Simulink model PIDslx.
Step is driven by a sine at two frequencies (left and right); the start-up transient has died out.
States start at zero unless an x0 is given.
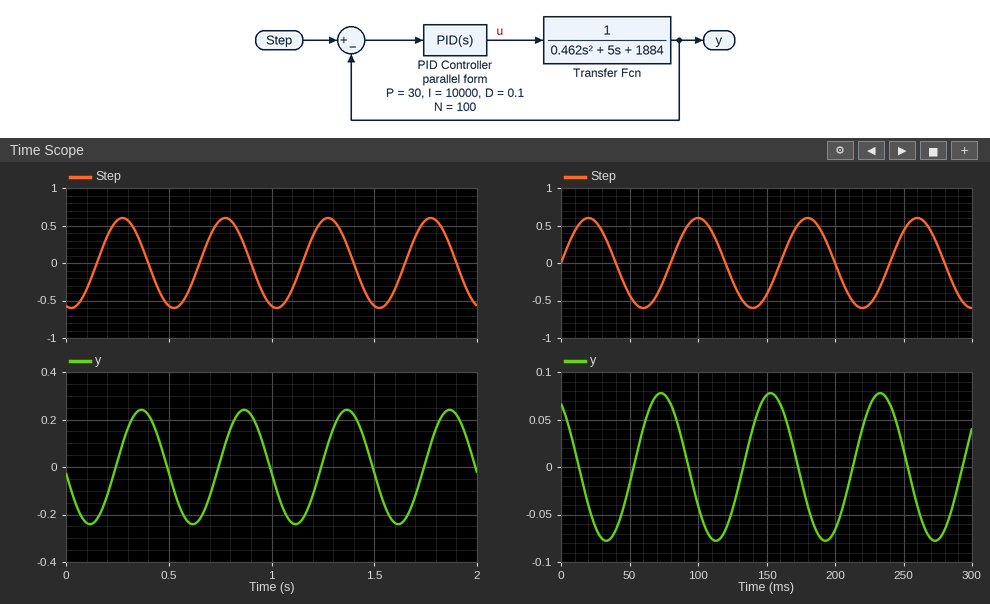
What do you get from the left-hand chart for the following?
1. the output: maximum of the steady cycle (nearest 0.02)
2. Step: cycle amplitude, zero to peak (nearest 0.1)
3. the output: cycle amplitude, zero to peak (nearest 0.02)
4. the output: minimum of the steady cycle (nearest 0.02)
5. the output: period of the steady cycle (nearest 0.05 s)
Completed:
0.24
0.6
0.24
-0.24
0.50 s
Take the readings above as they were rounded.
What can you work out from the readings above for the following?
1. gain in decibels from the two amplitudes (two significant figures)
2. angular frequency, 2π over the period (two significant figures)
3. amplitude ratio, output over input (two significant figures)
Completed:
-8.0 dB
13 rad/s
0.40
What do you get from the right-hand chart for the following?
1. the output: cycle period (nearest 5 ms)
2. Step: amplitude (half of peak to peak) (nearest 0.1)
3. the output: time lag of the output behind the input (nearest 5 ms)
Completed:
80 ms
0.6
55 ms
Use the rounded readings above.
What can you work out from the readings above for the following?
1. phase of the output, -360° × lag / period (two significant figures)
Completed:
-250°
